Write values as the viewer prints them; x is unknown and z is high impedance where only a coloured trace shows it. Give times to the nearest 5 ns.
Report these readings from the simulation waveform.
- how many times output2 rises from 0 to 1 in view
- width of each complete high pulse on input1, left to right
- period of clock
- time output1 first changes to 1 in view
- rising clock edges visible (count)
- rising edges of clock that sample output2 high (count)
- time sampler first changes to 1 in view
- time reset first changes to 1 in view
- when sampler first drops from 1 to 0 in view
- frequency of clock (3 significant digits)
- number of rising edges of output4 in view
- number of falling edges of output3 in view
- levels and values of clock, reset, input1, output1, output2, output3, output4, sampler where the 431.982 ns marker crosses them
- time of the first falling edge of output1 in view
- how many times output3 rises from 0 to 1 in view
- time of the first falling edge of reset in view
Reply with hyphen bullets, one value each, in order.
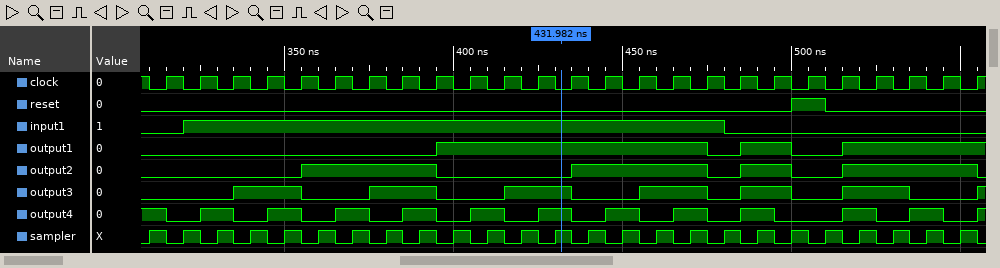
- 4
- 160 ns
- 10 ns
- 395 ns
- 25
- 13
- 310 ns
- 500 ns
- 315 ns
- 100 MHz
- 12
- 6
- clock=0, reset=0, input1=1, output1=1, output2=0, output3=1, output4=1, sampler=1
- 475 ns
- 7
- 510 ns
